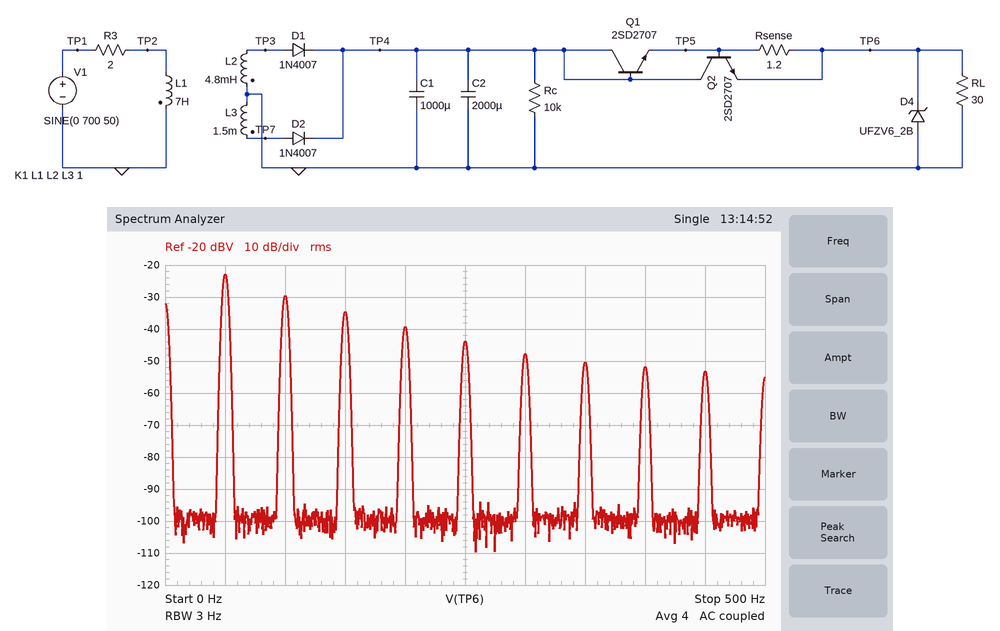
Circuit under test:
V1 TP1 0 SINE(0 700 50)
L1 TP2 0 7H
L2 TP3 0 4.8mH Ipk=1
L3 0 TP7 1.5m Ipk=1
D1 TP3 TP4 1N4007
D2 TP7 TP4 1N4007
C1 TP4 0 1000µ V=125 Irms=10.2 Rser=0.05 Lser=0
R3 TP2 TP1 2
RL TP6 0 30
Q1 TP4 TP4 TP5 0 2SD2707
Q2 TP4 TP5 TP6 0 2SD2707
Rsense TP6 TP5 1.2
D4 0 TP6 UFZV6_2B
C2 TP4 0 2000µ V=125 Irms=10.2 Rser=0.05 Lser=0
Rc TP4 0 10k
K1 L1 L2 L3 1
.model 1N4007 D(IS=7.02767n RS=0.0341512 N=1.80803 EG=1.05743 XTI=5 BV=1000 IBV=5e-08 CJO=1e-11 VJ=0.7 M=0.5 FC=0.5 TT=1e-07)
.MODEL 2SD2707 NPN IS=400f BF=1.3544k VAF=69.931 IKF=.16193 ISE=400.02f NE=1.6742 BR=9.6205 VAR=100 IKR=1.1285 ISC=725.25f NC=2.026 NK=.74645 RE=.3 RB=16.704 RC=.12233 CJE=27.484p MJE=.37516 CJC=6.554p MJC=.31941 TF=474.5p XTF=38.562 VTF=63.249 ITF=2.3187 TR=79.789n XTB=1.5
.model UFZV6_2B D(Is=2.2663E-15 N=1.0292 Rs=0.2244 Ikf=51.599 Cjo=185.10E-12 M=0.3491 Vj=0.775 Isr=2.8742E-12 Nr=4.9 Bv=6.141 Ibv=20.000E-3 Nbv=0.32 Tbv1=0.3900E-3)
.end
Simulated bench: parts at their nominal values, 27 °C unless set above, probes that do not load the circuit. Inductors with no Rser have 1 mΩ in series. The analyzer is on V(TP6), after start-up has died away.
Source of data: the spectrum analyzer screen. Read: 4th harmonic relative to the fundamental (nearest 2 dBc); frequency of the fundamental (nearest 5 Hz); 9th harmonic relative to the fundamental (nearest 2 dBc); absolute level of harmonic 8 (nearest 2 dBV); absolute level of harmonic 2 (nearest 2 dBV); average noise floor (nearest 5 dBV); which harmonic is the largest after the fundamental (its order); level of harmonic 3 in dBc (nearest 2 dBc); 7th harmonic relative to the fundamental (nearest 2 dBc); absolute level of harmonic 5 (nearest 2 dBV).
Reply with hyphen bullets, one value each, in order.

- -16 dBc
- 50 Hz
- -30 dBc
- -52 dBV
- -30 dBV
- -100 dBV
- 2
- -12 dBc
- -28 dBc
- -44 dBV
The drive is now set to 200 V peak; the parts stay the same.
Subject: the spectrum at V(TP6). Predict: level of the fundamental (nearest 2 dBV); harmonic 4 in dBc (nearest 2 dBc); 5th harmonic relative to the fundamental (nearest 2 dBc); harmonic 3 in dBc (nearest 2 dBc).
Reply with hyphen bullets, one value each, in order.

- -16 dBV
- -14 dBc
- -16 dBc
- -10 dBc
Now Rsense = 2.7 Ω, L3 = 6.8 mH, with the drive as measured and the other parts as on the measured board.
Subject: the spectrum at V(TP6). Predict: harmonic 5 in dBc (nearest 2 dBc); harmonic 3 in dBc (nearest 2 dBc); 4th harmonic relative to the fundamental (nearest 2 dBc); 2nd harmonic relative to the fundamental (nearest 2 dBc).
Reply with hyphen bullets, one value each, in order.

- -16 dBc
- -10 dBc
- -10 dBc
- 0 dBc
